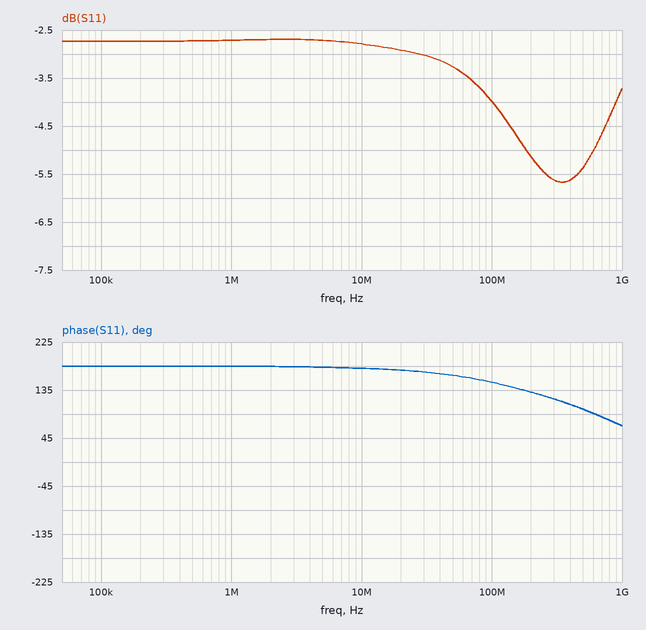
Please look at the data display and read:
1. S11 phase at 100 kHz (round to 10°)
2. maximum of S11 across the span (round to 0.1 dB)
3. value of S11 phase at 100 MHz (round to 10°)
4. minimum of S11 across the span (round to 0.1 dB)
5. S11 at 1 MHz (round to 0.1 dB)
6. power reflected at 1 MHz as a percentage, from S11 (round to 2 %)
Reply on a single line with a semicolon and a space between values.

180°; -2.7 dB; 150°; -5.7 dB; -2.7 dB; 54 %
